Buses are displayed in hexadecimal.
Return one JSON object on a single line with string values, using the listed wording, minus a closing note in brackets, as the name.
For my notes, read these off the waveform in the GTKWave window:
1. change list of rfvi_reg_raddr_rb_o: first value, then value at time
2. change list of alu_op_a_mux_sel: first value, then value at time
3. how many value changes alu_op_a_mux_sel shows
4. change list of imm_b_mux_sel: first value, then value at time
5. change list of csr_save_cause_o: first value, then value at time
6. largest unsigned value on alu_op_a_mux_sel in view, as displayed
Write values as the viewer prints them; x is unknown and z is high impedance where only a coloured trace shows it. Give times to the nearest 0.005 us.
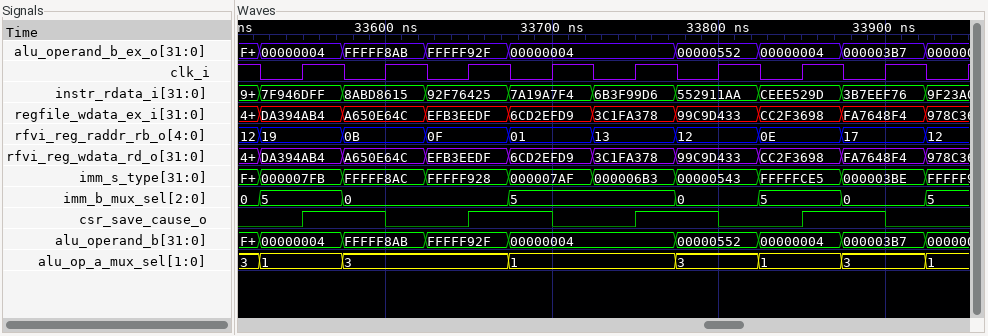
{"change list of rfvi_reg_raddr_rb_o: first value, then value at time": "12, 19 at 33.525 us, 0B at 33.575 us, 0F at 33.625 us, 01 at 33.675 us, 13 at 33.725 us, 12 at 33.775 us, 0E at 33.825 us, 17 at 33.875 us, 12 at 33.925 us", "change list of alu_op_a_mux_sel: first value, then value at time": "3, 1 at 33.525 us, 3 at 33.575 us, 1 at 33.675 us, 3 at 33.775 us, 1 at 33.825 us, 3 at 33.875 us, 1 at 33.925 us", "how many value changes alu_op_a_mux_sel shows": "7", "change list of imm_b_mux_sel: first value, then value at time": "0, 5 at 33.525 us, 0 at 33.575 us, 5 at 33.675 us, 0 at 33.775 us, 5 at 33.825 us, 0 at 33.875 us, 5 at 33.925 us", "change list of csr_save_cause_o: first value, then value at time": "0, 1 at 33.55 us, 0 at 33.6 us, 1 at 33.65 us, 0 at 33.7 us, 1 at 33.75 us, 0 at 33.8 us, 1 at 33.85 us, 0 at 33.9 us", "largest unsigned value on alu_op_a_mux_sel in view, as displayed": "3"}
